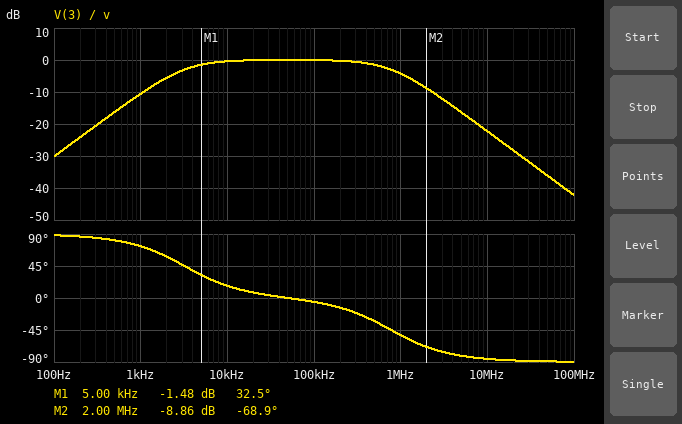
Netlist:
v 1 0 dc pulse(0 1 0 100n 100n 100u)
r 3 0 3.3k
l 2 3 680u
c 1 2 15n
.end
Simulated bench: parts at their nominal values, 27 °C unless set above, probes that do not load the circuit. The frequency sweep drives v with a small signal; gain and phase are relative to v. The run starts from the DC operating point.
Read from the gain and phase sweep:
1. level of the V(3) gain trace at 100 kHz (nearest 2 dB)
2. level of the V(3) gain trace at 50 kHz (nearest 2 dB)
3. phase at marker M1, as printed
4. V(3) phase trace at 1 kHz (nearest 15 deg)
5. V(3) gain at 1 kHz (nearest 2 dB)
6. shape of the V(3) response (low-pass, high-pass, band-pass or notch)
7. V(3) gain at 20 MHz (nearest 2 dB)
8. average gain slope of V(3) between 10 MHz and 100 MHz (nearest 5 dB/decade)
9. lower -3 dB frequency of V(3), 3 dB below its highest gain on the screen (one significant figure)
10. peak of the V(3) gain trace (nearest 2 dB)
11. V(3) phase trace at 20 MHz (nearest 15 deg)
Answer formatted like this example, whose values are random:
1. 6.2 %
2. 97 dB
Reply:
1. 0 dB
2. 0 dB
3. 32.5 deg
4. 75 deg
5. -10 dB
6. band-pass
7. -28 dB
8. -20 dB/decade
9. 3 kHz
10. 0 dB
11. -90 deg
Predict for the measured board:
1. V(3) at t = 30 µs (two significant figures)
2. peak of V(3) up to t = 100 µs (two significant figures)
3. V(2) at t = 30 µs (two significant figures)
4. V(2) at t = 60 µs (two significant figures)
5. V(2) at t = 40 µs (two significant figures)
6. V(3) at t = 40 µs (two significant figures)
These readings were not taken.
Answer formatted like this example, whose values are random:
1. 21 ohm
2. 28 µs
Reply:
1. 550 mV
2. 980 mV
3. 550 mV
4. 300 mV
5. 450 mV
6. 450 mV
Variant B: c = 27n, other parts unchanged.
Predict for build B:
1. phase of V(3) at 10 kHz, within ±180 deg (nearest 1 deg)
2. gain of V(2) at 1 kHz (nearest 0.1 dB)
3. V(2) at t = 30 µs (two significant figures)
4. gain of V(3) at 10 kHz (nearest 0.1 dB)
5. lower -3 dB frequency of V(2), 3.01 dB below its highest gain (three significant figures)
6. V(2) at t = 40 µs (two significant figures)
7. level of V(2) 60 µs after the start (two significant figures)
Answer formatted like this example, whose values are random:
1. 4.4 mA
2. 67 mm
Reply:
1. 9 deg
2. -6.2 dB
3. 720 mV
4. -0.1 dB
5. 1.79 kHz
6. 640 mV
7. 510 mV
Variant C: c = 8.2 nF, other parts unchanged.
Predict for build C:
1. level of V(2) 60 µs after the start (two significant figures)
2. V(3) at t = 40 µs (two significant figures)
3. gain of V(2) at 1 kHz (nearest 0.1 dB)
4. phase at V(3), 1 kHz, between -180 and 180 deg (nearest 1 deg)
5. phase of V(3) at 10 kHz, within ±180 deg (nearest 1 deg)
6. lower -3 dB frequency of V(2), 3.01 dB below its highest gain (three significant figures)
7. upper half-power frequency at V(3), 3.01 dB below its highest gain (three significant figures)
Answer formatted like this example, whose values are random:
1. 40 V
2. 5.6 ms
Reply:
1. 110 mV
2. 230 mV
3. -15.5 dB
4. 80 deg
5. 30 deg
6. 5.92 kHz
7. 778 kHz
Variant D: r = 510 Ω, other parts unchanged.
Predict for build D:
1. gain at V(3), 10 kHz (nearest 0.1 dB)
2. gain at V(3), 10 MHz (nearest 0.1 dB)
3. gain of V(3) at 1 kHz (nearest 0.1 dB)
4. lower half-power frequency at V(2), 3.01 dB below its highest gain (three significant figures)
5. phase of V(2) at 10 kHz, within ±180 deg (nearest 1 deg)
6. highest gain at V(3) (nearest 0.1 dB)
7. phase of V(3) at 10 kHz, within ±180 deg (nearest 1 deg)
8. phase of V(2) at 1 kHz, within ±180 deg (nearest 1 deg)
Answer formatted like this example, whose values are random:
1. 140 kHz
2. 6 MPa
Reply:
1. -7.0 dB
2. -38.5 dB
3. -26.4 dB
4. 21.0 kHz
5. 68 deg
6. 0 dB
7. 63 deg
8. 88 deg
